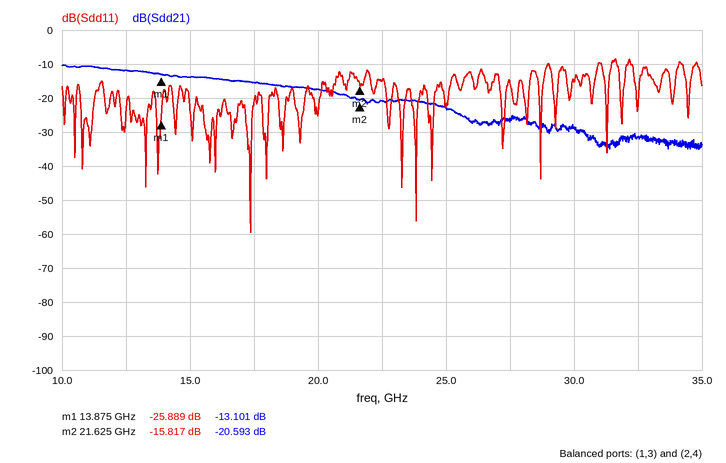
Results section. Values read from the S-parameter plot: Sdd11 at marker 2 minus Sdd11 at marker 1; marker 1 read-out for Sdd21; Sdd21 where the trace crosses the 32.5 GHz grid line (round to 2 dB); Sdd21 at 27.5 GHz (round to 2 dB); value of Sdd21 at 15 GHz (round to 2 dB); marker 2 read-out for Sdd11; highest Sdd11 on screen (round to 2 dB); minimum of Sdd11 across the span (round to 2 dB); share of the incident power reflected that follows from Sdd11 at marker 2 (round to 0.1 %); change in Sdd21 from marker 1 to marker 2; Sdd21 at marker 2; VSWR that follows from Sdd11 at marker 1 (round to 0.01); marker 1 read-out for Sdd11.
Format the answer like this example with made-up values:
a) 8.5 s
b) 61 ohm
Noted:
a) 10.072 dB
b) -13.101 dB
c) -32 dB
d) -26 dB
e) -14 dB
f) -15.817 dB
g) -8 dB
h) -60 dB
i) 2.6 %
j) -7.492 dB
k) -20.593 dB
l) 1.11
m) -25.889 dB
